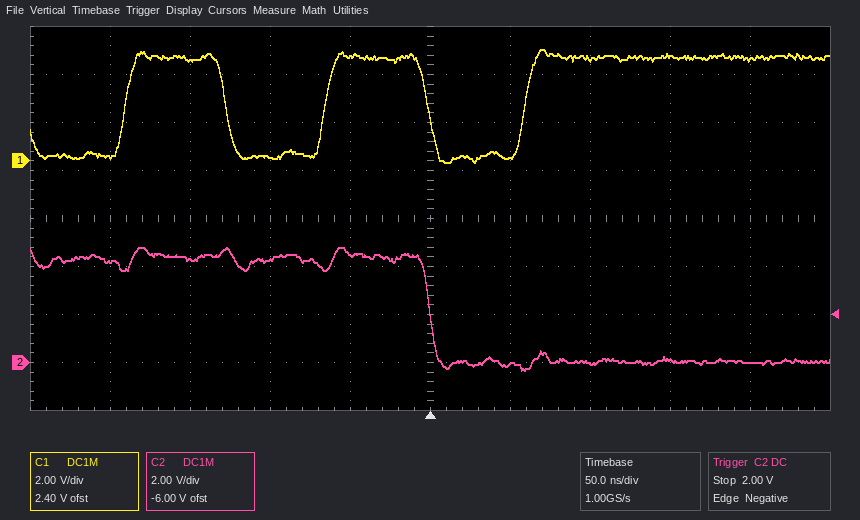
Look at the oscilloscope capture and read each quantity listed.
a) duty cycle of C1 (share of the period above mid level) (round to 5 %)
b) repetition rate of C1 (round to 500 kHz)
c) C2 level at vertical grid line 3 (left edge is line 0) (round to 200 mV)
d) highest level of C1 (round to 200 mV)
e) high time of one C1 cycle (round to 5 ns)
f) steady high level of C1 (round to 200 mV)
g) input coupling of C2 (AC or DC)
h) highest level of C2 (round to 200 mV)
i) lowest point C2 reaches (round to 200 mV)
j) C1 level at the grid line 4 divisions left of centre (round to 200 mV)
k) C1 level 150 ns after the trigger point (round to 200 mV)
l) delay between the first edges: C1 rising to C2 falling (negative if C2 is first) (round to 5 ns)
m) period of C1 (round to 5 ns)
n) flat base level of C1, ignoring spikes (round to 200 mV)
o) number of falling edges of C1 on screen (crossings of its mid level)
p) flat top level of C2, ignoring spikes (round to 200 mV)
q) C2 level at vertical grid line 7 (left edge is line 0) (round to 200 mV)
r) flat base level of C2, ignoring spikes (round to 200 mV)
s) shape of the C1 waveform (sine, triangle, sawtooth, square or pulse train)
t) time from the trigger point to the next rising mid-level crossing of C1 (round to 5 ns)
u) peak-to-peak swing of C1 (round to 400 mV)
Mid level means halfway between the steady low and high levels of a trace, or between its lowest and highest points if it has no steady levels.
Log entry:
50 %
8.0 MHz
4.4 V
4.6 V
65 ns
4.4 V
DC
4.8 V
-400 mV
200 mV
4.4 V
+190 ns
125 ns
200 mV
2
4.4 V
0.0 V
0.0 V
square
60 ns
4.8 V
